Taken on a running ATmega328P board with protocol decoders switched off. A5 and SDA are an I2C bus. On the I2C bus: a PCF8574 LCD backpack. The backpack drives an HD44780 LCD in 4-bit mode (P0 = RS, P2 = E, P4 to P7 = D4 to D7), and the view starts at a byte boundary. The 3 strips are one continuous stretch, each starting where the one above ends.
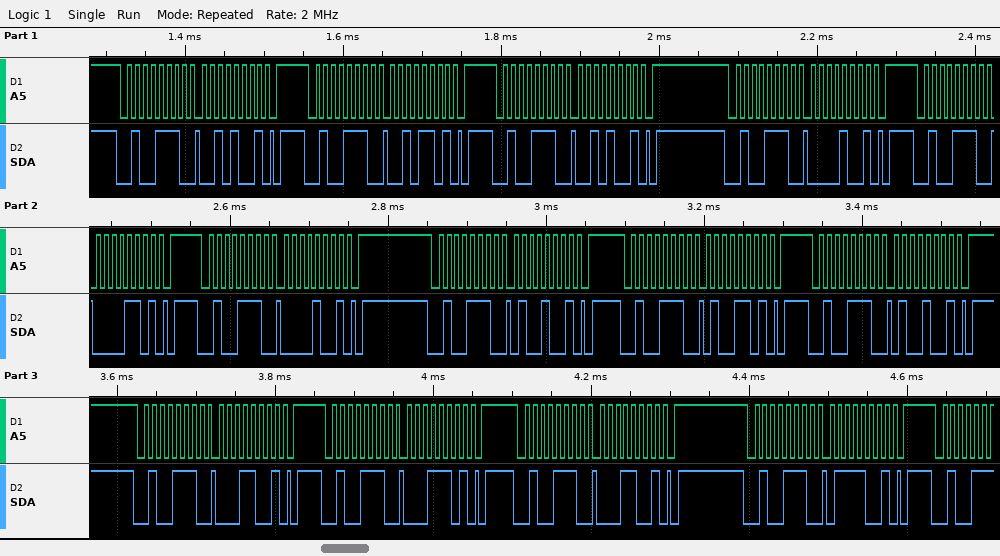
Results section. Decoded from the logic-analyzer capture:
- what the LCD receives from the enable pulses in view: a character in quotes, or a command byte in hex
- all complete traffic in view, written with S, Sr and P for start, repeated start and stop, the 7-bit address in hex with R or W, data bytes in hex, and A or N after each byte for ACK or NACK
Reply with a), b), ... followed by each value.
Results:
a) ' ' 'A'
b) S 27W A 29 A P S 27W A 2D A P S 27W A 29 A P S 27W A 09 A P S 27W A 0D A P S 27W A 09 A P S 27W A 49 A P S 27W A 4D A P S 27W A 49 A P S 27W A 19 A P S 27W A 1D A P S 27W A 19 A P S 27W A 79 A P
